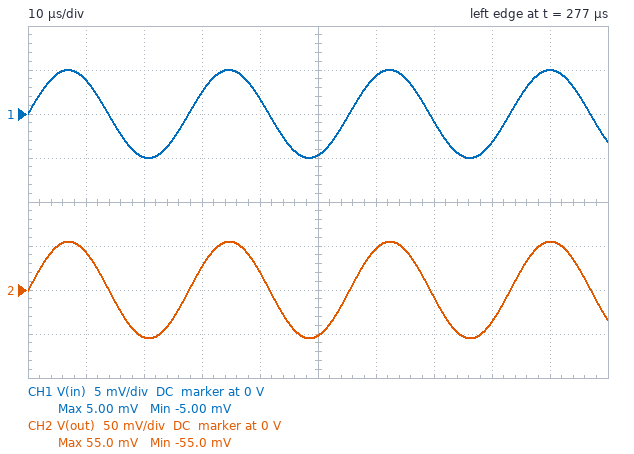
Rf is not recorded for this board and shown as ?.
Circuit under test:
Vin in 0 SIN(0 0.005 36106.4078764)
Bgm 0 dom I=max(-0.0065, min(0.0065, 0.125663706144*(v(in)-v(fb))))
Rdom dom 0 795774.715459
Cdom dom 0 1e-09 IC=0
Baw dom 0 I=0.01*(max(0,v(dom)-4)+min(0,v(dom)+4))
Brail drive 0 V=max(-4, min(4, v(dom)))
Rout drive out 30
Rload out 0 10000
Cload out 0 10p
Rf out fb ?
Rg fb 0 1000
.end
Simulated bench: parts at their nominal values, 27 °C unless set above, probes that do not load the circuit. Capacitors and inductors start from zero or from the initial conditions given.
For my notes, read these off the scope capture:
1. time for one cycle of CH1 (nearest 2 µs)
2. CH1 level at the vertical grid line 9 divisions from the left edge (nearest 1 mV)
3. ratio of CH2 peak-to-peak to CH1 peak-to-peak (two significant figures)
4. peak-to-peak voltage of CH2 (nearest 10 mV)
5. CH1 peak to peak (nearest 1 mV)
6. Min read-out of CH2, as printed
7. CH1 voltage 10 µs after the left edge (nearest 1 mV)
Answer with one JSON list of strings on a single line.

["28 µs", "5 mV", "11", "110 mV", "10 mV", "-55.0 mV", "4 mV"]
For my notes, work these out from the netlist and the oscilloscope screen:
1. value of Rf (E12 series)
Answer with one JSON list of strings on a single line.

["10 kΩ"]
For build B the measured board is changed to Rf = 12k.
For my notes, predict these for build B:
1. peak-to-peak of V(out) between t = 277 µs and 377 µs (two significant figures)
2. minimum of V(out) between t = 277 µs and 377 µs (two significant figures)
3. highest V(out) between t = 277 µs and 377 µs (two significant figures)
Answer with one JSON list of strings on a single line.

["130 mV", "-65 mV", "65 mV"]
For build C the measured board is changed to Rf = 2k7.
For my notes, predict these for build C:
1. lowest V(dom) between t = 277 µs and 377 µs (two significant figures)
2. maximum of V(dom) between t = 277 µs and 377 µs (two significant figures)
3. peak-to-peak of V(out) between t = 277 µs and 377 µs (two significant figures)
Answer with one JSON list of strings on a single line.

["-19 mV", "19 mV", "37 mV"]
